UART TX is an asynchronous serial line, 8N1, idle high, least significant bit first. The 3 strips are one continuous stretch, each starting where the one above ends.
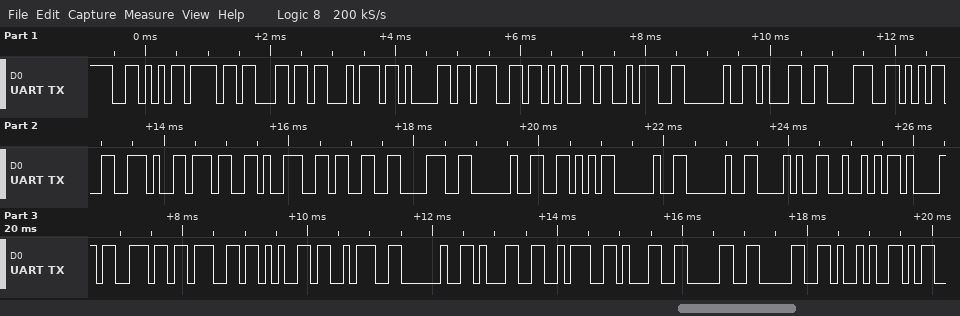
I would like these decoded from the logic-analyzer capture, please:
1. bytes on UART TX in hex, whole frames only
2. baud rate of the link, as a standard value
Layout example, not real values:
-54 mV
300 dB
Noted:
56 6F 6C 74 61 67 65 3A 20 31 38 35 2E 37 39 33 38 20 56 20 20 28 52 61 6E 67 65 3A 20 31 3A 31 30 30 29
9600 baud
